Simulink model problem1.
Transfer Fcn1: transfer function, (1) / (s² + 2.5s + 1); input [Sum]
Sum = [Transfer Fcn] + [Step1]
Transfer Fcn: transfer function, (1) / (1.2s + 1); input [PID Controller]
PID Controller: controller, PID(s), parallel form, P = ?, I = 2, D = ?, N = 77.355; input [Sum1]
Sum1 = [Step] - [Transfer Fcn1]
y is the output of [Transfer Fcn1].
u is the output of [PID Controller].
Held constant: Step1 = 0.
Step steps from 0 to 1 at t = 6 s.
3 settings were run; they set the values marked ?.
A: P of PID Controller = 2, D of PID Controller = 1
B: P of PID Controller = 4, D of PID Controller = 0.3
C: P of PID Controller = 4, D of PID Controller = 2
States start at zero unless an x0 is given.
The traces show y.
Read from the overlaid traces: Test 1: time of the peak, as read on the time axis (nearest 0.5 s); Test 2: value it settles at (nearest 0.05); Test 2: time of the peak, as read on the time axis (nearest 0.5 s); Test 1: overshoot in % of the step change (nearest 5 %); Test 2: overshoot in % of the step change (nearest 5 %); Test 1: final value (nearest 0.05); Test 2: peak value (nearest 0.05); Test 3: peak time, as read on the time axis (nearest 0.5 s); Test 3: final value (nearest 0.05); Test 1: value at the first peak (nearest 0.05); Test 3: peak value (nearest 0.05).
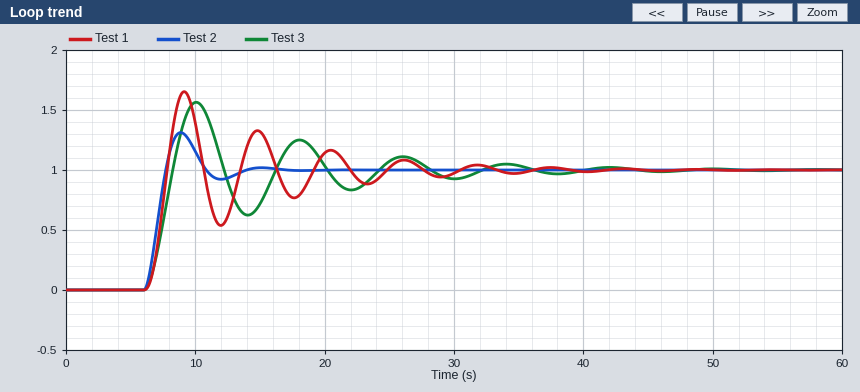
9.0 s
1.00
9.0 s
65 %
30 %
1.00
1.30
10.0 s
1.00
1.65
1.55
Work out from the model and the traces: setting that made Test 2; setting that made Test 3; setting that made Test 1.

C
A
B
